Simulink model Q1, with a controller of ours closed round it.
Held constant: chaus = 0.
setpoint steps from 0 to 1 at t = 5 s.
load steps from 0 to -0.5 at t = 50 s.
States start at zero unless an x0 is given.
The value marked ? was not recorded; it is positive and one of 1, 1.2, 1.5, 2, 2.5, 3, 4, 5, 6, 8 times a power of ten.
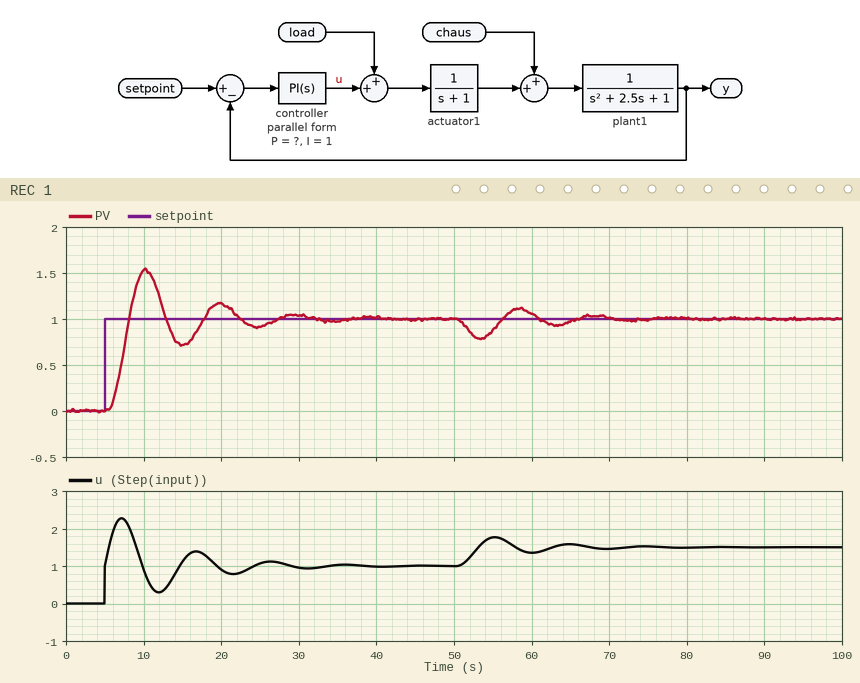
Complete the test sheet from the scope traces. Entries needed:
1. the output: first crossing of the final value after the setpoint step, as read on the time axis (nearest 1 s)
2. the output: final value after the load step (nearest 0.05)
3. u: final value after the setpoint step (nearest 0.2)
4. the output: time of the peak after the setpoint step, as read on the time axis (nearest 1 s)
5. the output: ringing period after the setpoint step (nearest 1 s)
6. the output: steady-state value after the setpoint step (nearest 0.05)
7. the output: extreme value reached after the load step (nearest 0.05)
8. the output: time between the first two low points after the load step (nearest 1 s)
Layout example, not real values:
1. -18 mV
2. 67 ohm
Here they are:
1. 8 s
2. 1.00
3. 1.0
4. 10 s
5. 10 s
6. 1.00
7. 0.80
8. 10 s
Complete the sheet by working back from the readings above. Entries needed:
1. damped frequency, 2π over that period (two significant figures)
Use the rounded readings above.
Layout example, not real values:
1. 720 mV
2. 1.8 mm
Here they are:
1. 0.63 rad/s
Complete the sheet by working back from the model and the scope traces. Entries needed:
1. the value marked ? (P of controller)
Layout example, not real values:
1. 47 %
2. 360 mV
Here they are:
1. 1
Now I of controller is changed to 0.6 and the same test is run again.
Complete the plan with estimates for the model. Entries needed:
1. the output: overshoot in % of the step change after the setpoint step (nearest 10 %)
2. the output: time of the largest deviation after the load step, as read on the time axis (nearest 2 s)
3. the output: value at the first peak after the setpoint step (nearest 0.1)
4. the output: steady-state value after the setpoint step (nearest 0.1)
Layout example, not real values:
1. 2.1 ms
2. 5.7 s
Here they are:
1. 20 %
2. 54 s
3. 1.2
4. 1.0
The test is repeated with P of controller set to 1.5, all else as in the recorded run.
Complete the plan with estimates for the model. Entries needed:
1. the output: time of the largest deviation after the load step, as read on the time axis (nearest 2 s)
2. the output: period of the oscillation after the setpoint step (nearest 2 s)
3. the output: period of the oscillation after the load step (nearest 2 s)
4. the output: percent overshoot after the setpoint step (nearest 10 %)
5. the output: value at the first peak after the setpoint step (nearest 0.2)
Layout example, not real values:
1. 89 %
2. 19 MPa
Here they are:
1. 54 s
2. 8 s
3. 8 s
4. 40 %
5. 1.4
